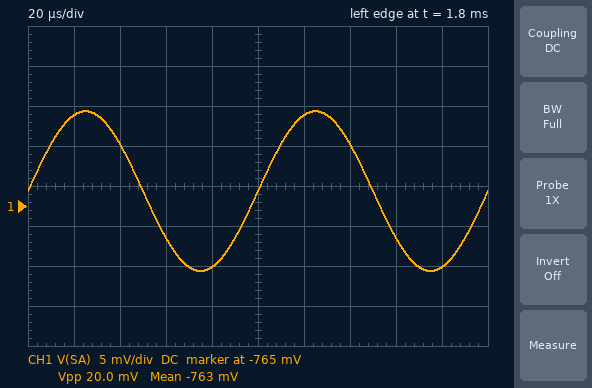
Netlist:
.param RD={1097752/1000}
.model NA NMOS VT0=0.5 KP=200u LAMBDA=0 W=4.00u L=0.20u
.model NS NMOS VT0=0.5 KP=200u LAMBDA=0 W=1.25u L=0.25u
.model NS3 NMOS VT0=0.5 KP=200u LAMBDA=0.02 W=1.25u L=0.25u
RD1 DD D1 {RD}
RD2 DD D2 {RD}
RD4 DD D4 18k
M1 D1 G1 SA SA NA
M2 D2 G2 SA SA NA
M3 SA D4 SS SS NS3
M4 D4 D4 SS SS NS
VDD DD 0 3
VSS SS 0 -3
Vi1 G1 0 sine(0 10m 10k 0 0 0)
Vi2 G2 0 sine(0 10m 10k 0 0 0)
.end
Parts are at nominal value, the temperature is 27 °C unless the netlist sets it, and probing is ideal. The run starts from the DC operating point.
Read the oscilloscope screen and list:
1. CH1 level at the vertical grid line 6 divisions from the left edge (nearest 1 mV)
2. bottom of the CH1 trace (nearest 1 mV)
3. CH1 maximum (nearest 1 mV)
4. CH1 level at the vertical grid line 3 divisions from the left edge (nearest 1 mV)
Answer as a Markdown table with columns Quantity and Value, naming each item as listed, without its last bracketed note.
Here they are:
| Quantity | Value |
|---|---|
| CH1 level at the vertical grid line 6 divisions from the left edge | -754 mV |
| bottom of the CH1 trace | -773 mV |
| CH1 maximum | -753 mV |
| CH1 level at the vertical grid line 3 divisions from the left edge | -769 mV |
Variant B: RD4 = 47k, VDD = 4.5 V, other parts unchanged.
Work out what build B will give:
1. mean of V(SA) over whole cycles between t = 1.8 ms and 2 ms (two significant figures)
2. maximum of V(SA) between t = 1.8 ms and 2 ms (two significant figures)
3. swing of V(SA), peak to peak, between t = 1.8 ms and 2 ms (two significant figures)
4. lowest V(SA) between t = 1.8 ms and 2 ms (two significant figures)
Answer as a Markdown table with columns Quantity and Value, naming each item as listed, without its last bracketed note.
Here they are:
| Quantity | Value |
|---|---|
| mean of V(SA) over whole cycles between t = 1.8 ms and 2 ms | -690 mV |
| maximum of V(SA) between t = 1.8 ms and 2 ms | -680 mV |
| swing of V(SA), peak to peak, between t = 1.8 ms and 2 ms | 20 mV |
| lowest V(SA) between t = 1.8 ms and 2 ms | -700 mV |
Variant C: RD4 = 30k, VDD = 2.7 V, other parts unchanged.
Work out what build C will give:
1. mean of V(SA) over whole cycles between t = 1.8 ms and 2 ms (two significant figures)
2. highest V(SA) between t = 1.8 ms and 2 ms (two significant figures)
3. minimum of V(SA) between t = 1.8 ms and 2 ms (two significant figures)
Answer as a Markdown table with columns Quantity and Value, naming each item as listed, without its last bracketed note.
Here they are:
| Quantity | Value |
|---|---|
| mean of V(SA) over whole cycles between t = 1.8 ms and 2 ms | -700 mV |
| highest V(SA) between t = 1.8 ms and 2 ms | -690 mV |
| minimum of V(SA) between t = 1.8 ms and 2 ms | -710 mV |
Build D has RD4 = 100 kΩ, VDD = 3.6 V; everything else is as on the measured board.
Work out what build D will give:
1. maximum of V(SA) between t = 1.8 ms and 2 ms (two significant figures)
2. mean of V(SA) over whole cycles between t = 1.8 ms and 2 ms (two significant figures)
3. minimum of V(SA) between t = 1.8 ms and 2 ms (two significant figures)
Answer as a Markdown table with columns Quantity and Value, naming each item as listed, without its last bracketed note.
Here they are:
| Quantity | Value |
|---|---|
| maximum of V(SA) between t = 1.8 ms and 2 ms | -610 mV |
| mean of V(SA) over whole cycles between t = 1.8 ms and 2 ms | -620 mV |
| minimum of V(SA) between t = 1.8 ms and 2 ms | -630 mV |
